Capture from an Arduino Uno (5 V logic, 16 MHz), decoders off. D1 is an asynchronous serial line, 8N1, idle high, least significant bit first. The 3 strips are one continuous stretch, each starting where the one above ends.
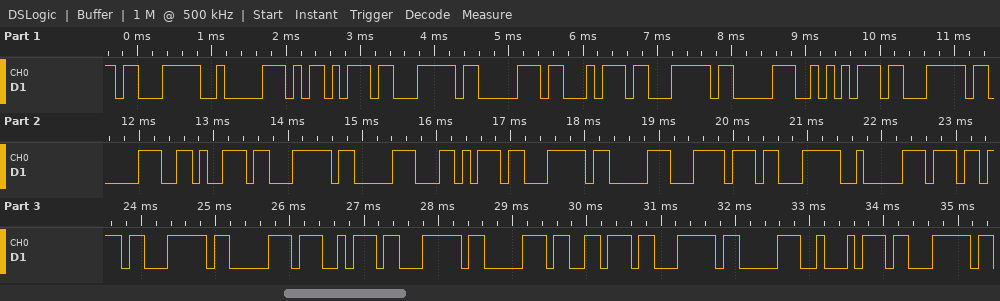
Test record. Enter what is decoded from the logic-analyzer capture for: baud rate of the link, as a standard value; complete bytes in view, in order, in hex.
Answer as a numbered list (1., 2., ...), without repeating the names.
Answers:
1. 9600 baud
2. E3 82 AD E3 83 A3 E3 83 AA E3 83 96 E3 83 AC E3 83 BC E3 82 B7 E3 83 A7 E3 83 B3 E3 83 A2 E3
